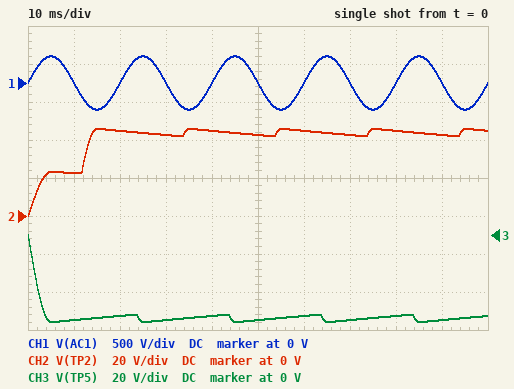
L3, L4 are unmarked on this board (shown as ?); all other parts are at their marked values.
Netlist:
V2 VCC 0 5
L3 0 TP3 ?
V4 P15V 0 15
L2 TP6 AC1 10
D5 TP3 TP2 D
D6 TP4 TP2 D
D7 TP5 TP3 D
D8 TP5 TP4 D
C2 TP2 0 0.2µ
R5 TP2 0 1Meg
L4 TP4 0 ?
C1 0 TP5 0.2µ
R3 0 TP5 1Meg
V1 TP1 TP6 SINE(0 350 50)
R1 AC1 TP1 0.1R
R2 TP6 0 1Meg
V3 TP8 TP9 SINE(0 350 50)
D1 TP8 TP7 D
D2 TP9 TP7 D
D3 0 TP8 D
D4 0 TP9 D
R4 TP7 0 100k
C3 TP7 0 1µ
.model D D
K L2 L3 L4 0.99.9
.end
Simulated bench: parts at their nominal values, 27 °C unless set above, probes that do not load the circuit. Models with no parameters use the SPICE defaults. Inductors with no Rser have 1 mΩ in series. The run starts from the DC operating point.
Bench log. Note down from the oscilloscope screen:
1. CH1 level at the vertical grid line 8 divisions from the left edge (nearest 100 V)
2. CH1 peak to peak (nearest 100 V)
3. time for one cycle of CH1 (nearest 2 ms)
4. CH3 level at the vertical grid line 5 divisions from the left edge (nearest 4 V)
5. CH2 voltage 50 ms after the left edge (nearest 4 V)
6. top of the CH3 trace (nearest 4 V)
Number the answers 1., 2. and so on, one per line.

1. 0 V
2. 700 V
3. 20 ms
4. -44 V
5. 44 V
6. 0 V
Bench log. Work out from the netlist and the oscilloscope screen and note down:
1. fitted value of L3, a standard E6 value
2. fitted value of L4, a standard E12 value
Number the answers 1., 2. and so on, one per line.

1. 47 mH
2. 180 mH
